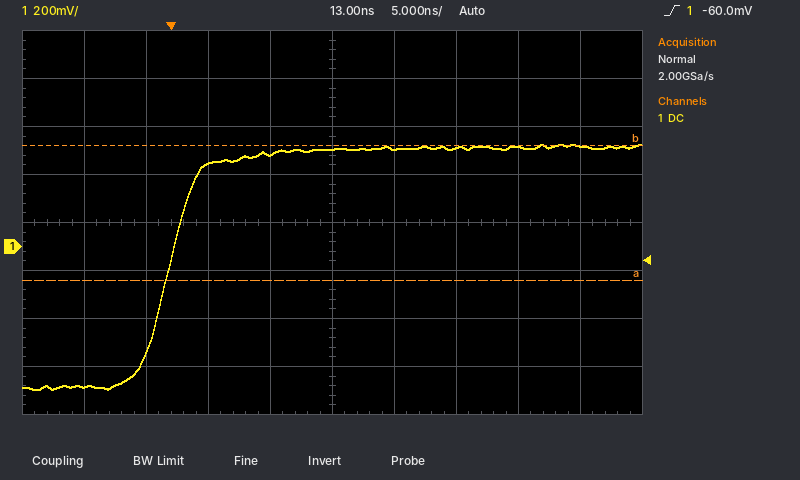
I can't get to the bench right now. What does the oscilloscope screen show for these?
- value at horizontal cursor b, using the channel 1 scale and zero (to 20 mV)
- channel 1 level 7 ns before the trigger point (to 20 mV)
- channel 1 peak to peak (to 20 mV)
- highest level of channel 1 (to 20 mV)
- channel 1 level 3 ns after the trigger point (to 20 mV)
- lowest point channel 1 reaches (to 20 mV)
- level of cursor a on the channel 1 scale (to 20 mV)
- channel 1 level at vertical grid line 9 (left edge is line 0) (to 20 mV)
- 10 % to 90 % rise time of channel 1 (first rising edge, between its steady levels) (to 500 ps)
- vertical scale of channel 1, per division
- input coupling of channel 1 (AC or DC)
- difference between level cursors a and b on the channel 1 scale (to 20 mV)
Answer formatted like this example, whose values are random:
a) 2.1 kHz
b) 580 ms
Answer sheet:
a) 420 mV
b) -580 mV
c) 1.02 V
d) 420 mV
e) 340 mV
f) -600 mV
g) -140 mV
h) 420 mV
i) 4.5 ns
j) 200 mV
k) DC
l) 560 mV
